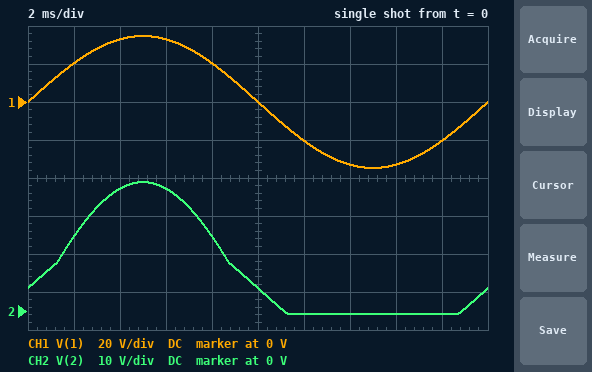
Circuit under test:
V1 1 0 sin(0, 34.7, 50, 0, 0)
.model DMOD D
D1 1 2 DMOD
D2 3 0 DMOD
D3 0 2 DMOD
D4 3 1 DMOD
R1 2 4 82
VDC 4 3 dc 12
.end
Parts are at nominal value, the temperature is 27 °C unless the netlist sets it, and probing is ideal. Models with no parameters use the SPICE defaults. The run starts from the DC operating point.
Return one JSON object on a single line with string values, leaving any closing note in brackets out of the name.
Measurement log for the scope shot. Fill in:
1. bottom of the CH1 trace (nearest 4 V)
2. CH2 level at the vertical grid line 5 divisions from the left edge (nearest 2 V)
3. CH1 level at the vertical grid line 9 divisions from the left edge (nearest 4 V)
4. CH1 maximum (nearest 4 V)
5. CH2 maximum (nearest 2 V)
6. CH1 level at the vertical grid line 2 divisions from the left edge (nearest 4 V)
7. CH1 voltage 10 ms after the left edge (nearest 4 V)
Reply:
{"bottom of the CH1 trace": "-36 V", "CH2 level at the vertical grid line 5 divisions from the left edge": "6 V", "CH1 level at the vertical grid line 9 divisions from the left edge": "-20 V", "CH1 maximum": "36 V", "CH2 maximum": "34 V", "CH1 level at the vertical grid line 2 divisions from the left edge": "32 V", "CH1 voltage 10 ms after the left edge": "0 V"}
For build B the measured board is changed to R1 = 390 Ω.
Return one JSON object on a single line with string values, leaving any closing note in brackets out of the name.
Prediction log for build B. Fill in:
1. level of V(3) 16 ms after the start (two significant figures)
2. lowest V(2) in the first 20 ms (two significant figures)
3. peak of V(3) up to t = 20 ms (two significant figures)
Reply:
{"level of V(3) 16 ms after the start": "-32 V", "lowest V(2) in the first 20 ms": "-760 mV", "peak of V(3) up to t = 20 ms": "760 mV"}
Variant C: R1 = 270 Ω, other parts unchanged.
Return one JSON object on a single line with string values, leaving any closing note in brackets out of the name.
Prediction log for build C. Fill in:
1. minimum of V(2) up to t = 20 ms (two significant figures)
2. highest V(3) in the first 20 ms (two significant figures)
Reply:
{"minimum of V(2) up to t = 20 ms": "-770 mV", "highest V(3) in the first 20 ms": "770 mV"}
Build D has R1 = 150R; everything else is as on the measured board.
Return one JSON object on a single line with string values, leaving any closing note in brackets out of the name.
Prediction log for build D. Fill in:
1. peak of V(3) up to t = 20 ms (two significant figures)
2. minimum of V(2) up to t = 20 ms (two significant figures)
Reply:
{"peak of V(3) up to t = 20 ms": "780 mV", "minimum of V(2) up to t = 20 ms": "-780 mV"}
